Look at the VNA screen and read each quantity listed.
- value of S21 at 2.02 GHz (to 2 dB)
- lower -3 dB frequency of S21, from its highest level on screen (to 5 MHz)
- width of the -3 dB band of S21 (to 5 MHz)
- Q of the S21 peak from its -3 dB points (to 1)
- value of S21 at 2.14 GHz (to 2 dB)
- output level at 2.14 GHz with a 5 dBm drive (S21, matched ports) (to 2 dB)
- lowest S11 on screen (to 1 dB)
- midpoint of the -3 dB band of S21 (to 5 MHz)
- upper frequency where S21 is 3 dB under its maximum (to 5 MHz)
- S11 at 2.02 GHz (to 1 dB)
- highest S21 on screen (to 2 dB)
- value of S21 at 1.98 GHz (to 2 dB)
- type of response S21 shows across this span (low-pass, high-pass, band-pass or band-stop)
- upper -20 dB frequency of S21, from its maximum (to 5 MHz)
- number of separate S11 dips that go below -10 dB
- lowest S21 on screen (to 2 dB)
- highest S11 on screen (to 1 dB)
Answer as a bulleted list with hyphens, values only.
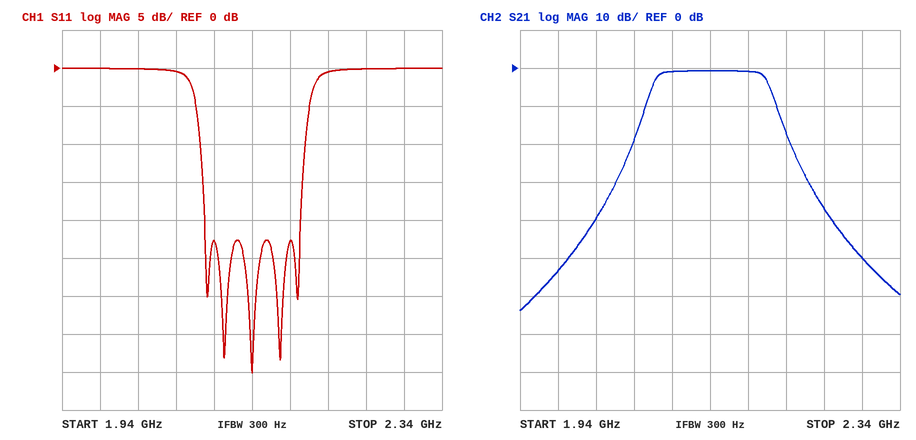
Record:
- -40 dB
- 2.080 GHz
- 120 MHz
- 18
- 0 dB
- 4 dBm
- -40 dB
- 2.140 GHz
- 2.200 GHz
- 0 dB
- 0 dB
- -54 dB
- band-pass
- 2.225 GHz
- 5
- -64 dB
- 0 dB
